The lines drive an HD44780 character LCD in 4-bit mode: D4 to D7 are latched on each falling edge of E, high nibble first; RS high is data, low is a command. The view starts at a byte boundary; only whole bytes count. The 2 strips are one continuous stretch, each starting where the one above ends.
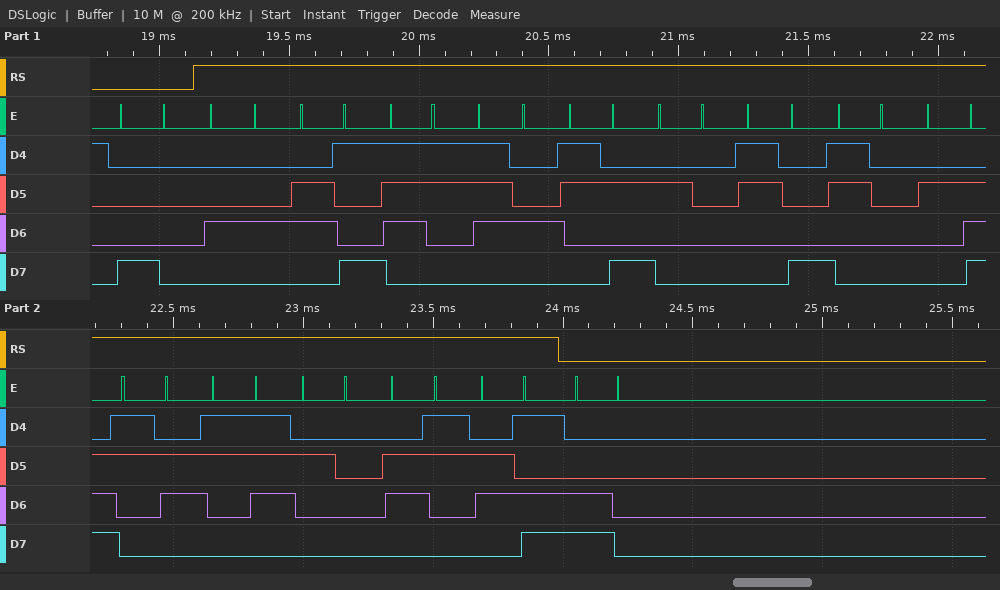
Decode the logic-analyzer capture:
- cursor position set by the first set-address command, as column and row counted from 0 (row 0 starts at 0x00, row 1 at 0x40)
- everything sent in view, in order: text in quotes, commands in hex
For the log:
column 0, row 0
0x80 "Dist: 80.67 cm" 0xC0
